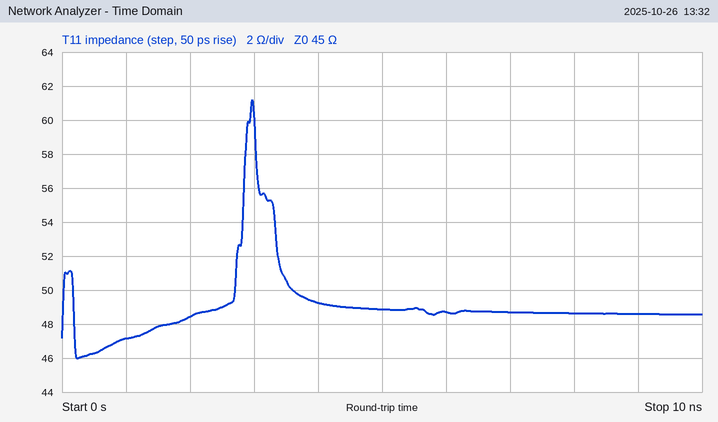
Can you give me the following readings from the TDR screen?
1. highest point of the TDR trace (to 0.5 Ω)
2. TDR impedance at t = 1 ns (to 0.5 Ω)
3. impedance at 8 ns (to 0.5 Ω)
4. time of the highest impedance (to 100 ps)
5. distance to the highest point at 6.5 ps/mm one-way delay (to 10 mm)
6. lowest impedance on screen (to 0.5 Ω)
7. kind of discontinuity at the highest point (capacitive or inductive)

61.0 Ω
47.0 Ω
48.5 Ω
3.0 ns
230 mm
46.0 Ω
inductive
